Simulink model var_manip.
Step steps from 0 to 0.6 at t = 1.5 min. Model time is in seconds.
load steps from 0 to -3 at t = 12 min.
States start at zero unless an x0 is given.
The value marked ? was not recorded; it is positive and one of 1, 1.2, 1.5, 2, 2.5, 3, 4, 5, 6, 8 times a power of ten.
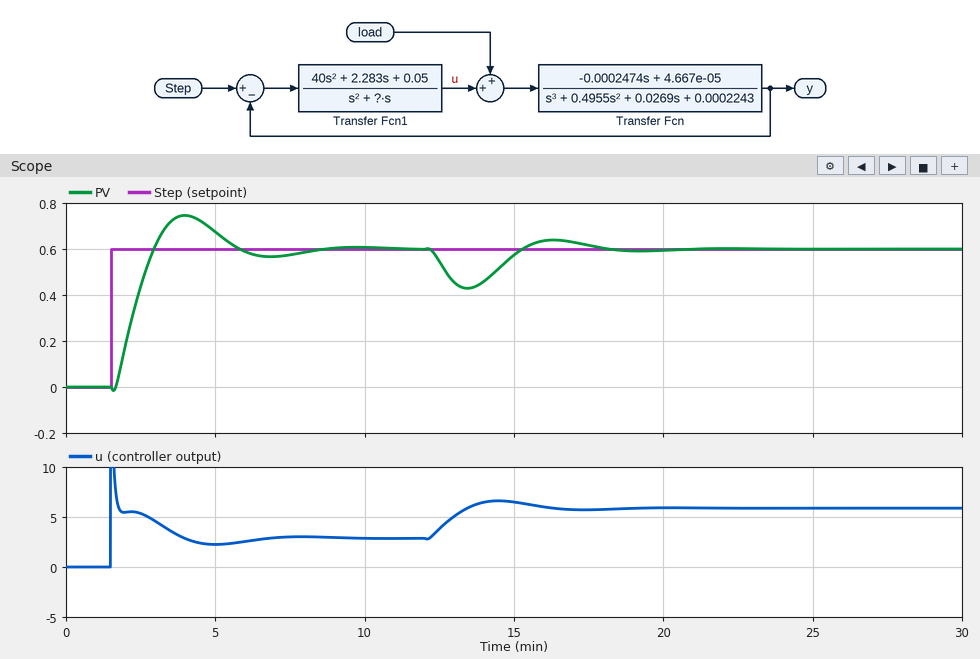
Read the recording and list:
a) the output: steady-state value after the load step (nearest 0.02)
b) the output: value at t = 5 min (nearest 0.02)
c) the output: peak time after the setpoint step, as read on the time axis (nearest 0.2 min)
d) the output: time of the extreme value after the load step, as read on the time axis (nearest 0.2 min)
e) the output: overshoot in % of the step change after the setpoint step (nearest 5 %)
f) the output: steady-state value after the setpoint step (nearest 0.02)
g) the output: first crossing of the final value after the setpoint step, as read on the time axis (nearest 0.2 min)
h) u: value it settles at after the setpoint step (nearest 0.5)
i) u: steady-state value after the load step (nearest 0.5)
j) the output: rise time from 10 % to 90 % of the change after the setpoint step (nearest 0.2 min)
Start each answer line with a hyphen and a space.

- 0.60
- 0.68
- 4.0 min
- 13.4 min
- 25 %
- 0.60
- 3.0 min
- 3.0
- 6.0
- 1.0 min
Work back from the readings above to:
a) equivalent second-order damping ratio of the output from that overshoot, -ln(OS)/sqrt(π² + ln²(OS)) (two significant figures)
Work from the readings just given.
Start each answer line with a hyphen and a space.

- 0.40
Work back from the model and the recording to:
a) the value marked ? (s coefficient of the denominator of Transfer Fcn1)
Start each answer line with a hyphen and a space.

- 0.25
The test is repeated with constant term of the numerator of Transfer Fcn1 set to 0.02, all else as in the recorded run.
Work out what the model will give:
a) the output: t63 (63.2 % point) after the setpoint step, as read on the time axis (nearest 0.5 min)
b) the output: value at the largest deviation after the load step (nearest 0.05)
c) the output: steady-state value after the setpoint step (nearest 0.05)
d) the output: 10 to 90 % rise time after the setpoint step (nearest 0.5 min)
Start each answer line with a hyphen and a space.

- 2.5 min
- 0.40
- 0.60
- 2.0 min
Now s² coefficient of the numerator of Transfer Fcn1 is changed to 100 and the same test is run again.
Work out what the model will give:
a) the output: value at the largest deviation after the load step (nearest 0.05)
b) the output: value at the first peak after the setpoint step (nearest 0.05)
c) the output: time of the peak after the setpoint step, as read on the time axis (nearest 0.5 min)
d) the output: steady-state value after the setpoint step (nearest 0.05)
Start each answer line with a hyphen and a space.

- 0.45
- 0.70
- 4.5 min
- 0.60
